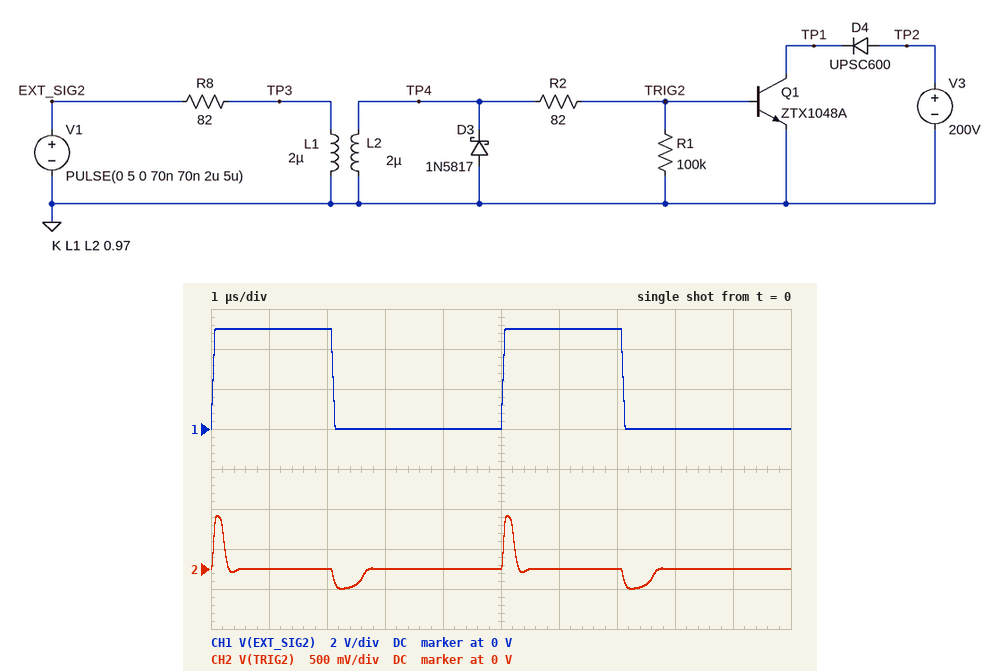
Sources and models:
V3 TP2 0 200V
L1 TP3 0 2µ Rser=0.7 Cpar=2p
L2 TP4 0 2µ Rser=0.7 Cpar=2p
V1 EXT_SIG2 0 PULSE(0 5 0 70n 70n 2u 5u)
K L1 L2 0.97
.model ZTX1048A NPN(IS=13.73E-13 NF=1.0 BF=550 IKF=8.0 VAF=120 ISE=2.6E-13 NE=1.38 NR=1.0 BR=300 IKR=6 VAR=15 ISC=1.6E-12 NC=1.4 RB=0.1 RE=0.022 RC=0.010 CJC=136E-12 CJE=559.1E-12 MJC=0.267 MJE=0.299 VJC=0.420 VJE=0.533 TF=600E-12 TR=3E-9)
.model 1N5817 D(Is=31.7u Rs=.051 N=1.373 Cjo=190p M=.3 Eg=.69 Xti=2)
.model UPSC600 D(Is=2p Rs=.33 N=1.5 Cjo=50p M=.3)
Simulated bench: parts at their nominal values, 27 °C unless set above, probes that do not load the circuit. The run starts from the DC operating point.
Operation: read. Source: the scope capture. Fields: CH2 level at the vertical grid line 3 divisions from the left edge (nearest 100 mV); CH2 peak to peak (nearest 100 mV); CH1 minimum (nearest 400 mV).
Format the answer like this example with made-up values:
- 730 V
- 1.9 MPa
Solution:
- 0 V
- 900 mV
- 0 V
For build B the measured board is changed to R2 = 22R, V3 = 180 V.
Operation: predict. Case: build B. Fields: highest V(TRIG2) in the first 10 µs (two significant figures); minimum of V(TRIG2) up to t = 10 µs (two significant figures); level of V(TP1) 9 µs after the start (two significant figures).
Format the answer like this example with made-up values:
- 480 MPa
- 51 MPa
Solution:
- 730 mV
- -260 mV
- 180 V
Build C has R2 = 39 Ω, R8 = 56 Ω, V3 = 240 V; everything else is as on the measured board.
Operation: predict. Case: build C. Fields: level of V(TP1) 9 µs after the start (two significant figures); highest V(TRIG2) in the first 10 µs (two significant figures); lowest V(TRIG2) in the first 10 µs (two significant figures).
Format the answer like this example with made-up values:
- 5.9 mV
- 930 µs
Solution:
- 240 V
- 740 mV
- -270 mV
